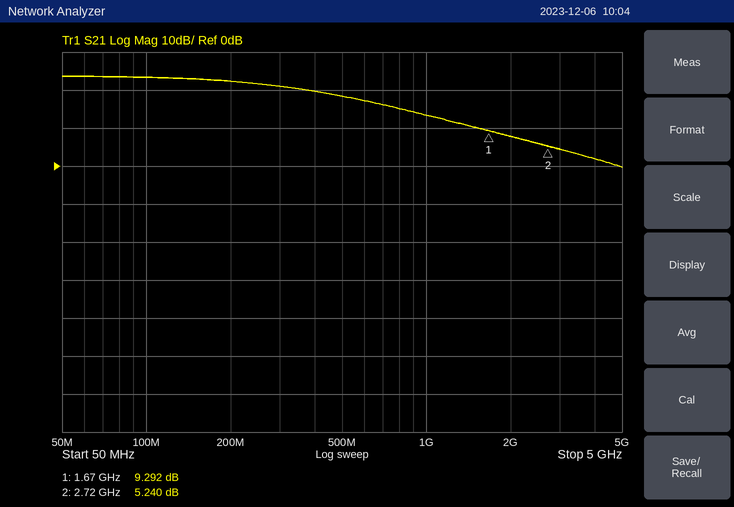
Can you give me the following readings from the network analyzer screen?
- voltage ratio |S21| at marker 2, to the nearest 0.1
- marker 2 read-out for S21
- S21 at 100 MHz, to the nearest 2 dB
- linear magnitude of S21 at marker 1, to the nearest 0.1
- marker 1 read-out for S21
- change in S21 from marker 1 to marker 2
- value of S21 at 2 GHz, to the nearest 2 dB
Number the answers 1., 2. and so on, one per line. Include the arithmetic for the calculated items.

1. 10^(5.24/20) ≈ 1.8
2. 5.240 dB
3. 24 dB
4. 10^(9.292/20) ≈ 2.9
5. 9.292 dB
6. 5.24 − (9.292) = -4.052 dB
7. 8 dB
